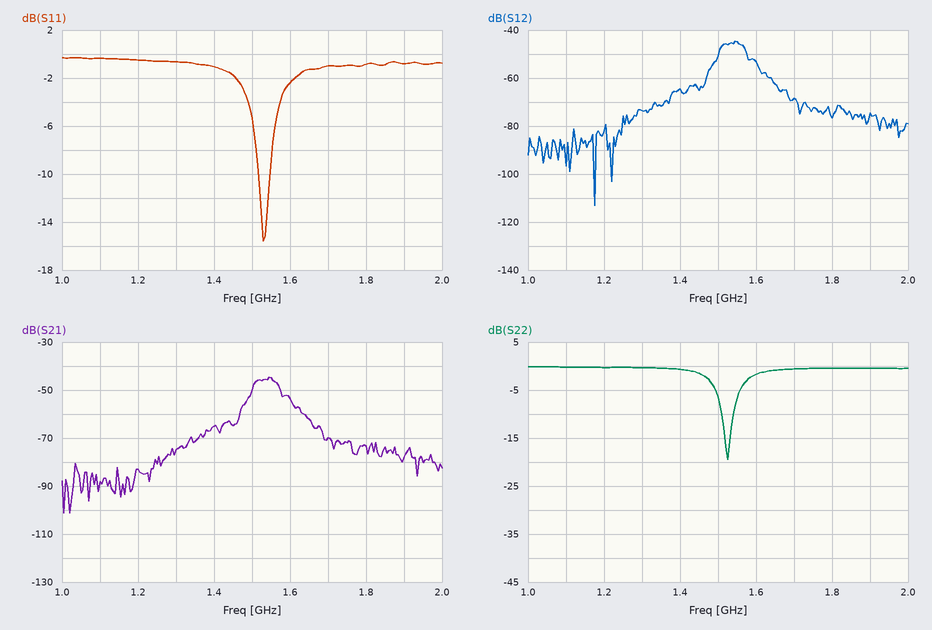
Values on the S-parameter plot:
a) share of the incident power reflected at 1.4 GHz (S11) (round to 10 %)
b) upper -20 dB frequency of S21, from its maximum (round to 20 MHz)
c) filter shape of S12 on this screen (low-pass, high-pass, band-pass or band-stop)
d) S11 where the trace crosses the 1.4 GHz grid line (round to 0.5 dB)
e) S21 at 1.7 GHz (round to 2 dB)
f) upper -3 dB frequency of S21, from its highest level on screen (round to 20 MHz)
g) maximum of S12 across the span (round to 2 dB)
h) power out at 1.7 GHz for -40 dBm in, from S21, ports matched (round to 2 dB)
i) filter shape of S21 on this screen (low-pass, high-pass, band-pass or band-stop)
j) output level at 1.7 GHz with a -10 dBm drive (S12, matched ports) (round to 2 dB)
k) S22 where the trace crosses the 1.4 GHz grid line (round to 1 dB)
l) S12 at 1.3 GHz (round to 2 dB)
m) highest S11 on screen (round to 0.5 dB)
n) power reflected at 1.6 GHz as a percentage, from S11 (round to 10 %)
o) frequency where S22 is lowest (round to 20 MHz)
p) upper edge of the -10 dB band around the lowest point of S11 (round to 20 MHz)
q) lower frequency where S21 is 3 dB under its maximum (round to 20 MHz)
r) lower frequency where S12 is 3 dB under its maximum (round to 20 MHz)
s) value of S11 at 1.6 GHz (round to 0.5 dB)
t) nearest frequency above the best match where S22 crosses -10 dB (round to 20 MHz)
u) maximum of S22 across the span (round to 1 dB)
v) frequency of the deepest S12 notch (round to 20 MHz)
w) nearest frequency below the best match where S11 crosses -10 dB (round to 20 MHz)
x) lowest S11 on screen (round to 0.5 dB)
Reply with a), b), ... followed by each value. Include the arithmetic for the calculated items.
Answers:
a) 10^(-1/10) ≈ 79.4 %, so 80 % to the nearest 10 %
b) 1.66 GHz
c) band-pass
d) -1.0 dB
e) -70 dB
f) 1.56 GHz
g) -44 dB
h) -40 dBm + (-70 dB) = -110 dBm
i) band-pass
j) -10 dBm + (-68 dB) = -78 dBm
k) -1 dB
l) -74 dB
m) -0.5 dB
n) 10^(-2.5/10) ≈ 56.2 %, so 60 % to the nearest 10 %
o) 1.52 GHz
p) 1.54 GHz
q) 1.50 GHz
r) 1.50 GHz
s) -2.5 dB
t) 1.54 GHz
u) 0 dB
v) 1.18 GHz
w) 1.52 GHz
x) -15.5 dB
